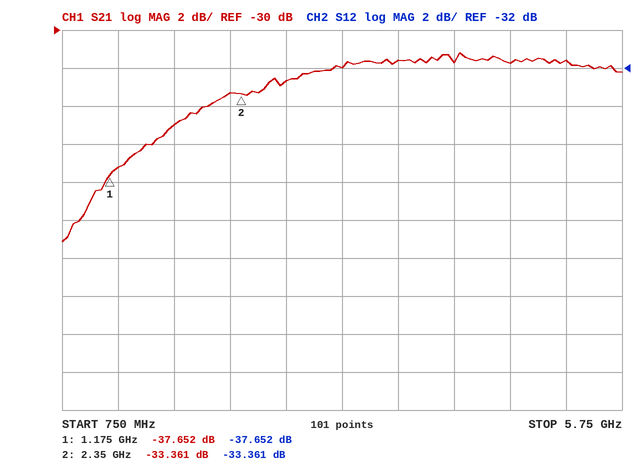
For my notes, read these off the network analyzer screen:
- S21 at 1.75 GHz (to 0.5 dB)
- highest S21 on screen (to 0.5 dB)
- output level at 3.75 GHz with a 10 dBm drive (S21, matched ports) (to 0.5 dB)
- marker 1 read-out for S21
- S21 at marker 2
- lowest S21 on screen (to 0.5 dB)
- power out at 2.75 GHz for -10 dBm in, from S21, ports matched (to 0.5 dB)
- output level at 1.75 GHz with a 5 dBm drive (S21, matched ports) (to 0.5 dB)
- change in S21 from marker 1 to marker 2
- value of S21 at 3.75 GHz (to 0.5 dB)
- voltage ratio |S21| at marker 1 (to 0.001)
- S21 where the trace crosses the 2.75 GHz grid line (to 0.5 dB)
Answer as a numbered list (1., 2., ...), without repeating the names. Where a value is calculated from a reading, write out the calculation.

1. -35.0 dB
2. -31.0 dB
3. 10 dBm + (-31.5 dB) = -21.5 dBm
4. -37.652 dB
5. -33.361 dB
6. -41.0 dB
7. -10 dBm + (-32.5 dB) = -42.5 dBm
8. 5 dBm + (-35.0 dB) = -30.0 dBm
9. -33.361 − (-37.652) = 4.291 dB
10. -31.5 dB
11. 10^(-37.652/20) ≈ 0.013
12. -32.5 dB
